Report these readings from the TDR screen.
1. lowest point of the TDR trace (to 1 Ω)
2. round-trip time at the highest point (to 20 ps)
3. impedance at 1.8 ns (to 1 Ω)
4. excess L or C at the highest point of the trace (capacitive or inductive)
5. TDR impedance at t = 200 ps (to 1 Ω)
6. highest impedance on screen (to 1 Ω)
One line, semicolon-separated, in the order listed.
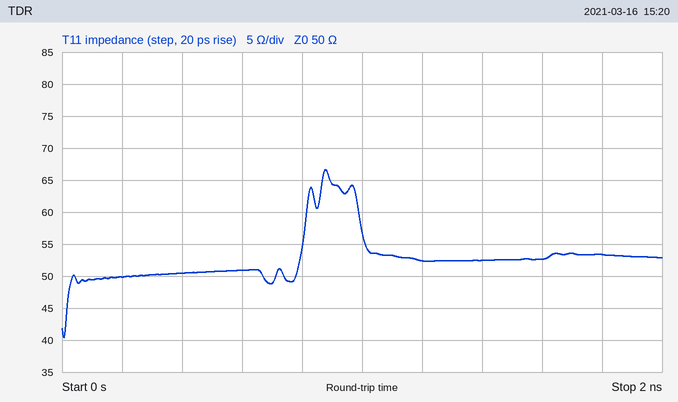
40 Ω; 880 ps; 53 Ω; inductive; 50 Ω; 67 Ω
